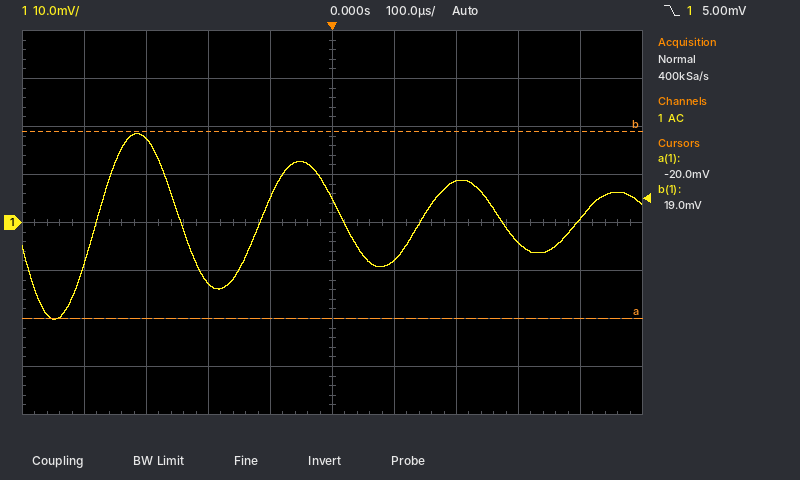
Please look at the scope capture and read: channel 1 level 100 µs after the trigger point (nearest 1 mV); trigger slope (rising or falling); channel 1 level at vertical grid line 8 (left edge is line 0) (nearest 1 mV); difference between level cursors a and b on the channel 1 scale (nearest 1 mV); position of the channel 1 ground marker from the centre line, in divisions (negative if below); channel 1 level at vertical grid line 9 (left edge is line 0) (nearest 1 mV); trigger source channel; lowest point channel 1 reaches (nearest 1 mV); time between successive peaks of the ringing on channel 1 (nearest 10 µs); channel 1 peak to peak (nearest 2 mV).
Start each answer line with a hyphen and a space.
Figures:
- -8 mV
- falling
- -4 mV
- 39 mV
- 0.0 div
- 1 mV
- channel 1
- -20 mV
- 260 µs
- 38 mV
